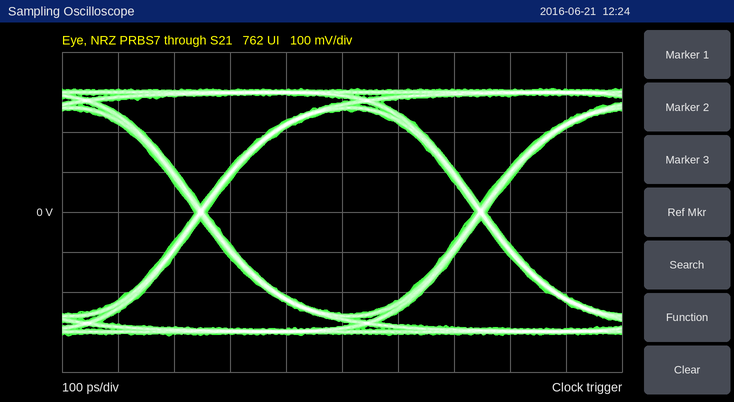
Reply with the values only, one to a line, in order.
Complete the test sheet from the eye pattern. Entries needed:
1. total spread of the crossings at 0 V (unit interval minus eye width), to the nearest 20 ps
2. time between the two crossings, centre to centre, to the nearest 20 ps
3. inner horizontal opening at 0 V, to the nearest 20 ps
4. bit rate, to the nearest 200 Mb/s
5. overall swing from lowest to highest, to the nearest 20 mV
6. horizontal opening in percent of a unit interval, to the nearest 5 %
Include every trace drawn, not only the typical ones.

20 ps
500 ps
480 ps
2.0 Gb/s
620 mV
95 %
